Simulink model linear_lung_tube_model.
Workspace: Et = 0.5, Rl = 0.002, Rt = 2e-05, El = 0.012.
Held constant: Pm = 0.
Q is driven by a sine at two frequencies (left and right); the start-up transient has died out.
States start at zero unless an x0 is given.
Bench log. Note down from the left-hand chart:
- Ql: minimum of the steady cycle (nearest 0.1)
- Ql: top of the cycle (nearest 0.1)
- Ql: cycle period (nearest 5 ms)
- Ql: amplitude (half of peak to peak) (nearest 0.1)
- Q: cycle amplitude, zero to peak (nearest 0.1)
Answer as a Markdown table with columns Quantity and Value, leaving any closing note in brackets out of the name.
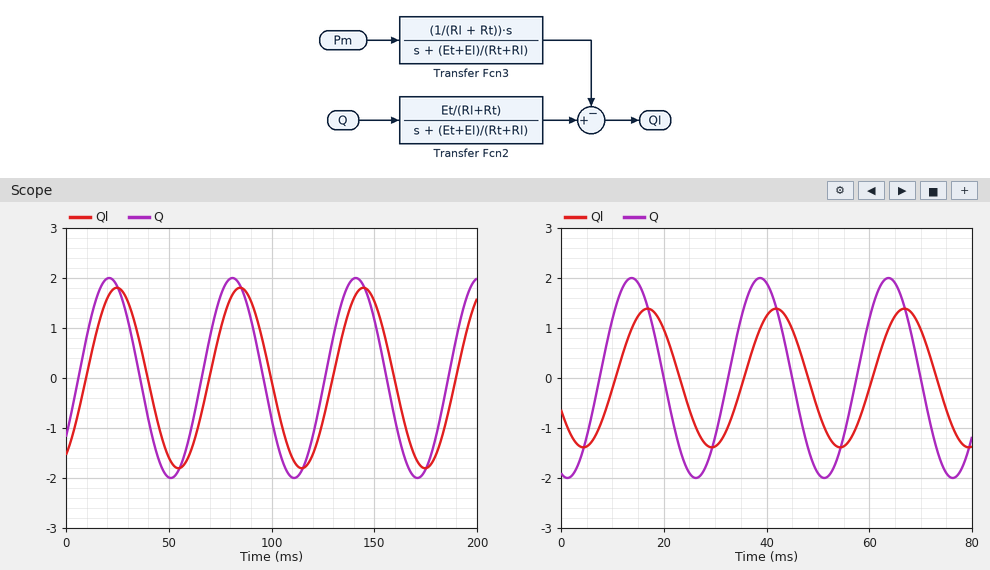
| Quantity | Value |
|---|---|
| Ql: minimum of the steady cycle | -1.8 |
| Ql: top of the cycle | 1.8 |
| Ql: cycle period | 60 ms |
| Ql: amplitude (half of peak to peak) | 1.8 |
| Q: cycle amplitude, zero to peak | 2.0 |
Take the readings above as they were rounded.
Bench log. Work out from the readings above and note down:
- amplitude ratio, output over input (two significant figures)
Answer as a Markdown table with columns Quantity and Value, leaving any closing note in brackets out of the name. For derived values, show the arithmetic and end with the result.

| Quantity | Value |
|---|---|
| amplitude ratio, output over input | 1.8 / 2 = 0.90 |
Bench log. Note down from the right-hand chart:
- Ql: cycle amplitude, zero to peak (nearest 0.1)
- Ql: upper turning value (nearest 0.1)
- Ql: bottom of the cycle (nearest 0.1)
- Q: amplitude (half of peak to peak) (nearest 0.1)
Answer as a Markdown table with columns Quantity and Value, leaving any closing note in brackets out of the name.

| Quantity | Value |
|---|---|
| Ql: cycle amplitude, zero to peak | 1.4 |
| Ql: upper turning value | 1.4 |
| Ql: bottom of the cycle | -1.4 |
| Q: amplitude (half of peak to peak) | 2.0 |
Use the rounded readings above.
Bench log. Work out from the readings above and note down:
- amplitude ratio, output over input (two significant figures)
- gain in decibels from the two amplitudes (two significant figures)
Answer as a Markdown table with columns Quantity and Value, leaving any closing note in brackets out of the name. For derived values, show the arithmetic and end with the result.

| Quantity | Value |
|---|---|
| amplitude ratio, output over input | 1.4 / 2 = 0.70 |
| gain in decibels from the two amplitudes | 20 log10(1.4 / 2) = -3.1 dB |
